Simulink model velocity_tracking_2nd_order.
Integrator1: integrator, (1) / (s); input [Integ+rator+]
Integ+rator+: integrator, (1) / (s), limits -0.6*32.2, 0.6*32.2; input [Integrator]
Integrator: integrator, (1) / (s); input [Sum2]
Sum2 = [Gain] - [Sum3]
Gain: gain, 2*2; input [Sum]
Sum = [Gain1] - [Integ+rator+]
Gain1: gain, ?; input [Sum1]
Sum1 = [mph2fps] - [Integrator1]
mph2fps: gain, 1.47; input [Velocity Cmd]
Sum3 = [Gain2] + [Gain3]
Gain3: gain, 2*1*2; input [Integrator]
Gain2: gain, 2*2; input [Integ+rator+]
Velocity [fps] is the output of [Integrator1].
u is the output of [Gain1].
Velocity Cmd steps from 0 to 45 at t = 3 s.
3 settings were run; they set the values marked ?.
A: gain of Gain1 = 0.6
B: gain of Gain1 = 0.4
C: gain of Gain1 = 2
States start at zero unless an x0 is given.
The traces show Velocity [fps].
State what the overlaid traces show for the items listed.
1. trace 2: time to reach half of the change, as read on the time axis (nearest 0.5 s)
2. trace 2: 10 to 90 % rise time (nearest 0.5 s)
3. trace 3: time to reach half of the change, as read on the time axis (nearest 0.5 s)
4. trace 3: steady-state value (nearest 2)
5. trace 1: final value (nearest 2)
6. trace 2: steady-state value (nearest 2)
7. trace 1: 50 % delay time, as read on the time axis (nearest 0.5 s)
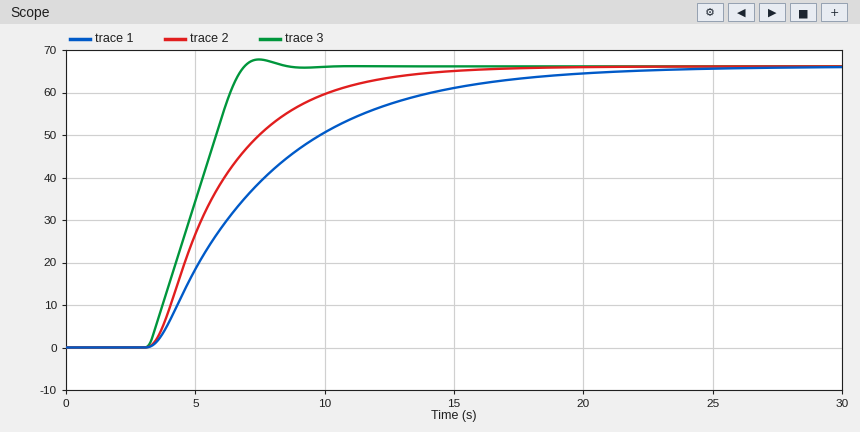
5.5 s
6.0 s
5.0 s
66
66
66
6.5 s
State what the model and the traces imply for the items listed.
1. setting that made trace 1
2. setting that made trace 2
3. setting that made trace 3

B
A
C
